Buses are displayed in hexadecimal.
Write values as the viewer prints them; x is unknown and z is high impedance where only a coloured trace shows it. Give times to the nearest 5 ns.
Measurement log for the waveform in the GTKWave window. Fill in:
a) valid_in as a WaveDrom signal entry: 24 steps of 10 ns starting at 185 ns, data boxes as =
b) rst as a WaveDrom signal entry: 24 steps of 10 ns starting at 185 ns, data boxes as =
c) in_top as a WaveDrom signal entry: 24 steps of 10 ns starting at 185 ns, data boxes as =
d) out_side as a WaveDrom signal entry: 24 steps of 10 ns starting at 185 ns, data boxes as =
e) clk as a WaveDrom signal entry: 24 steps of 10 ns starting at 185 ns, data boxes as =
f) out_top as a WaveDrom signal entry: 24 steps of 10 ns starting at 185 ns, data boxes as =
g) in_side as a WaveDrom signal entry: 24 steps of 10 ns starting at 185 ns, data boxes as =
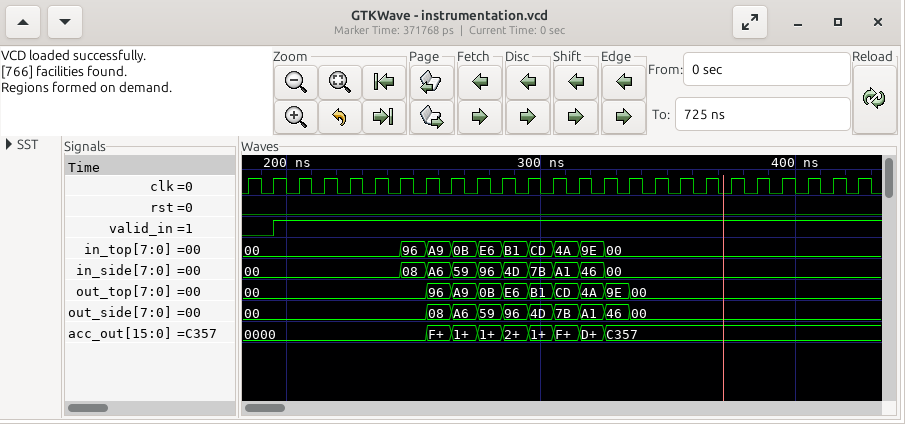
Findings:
{name: 'valid_in', wave: '01......................'}
{name: 'rst', wave: '0.......................'}
{name: 'in_top', wave: '=.....=========.........', data: '00 96 A9 0B E6 B1 CD 4A 9E 00'}
{name: 'out_side', wave: '=......=========........', data: '00 08 A6 59 96 4D 7B A1 46 00'}
{name: 'clk', wave: 'p.......................'}
{name: 'out_top', wave: '=......=========........', data: '00 96 A9 0B E6 B1 CD 4A 9E 00'}
{name: 'in_side', wave: '=.....=========.........', data: '00 08 A6 59 96 4D 7B A1 46 00'}
